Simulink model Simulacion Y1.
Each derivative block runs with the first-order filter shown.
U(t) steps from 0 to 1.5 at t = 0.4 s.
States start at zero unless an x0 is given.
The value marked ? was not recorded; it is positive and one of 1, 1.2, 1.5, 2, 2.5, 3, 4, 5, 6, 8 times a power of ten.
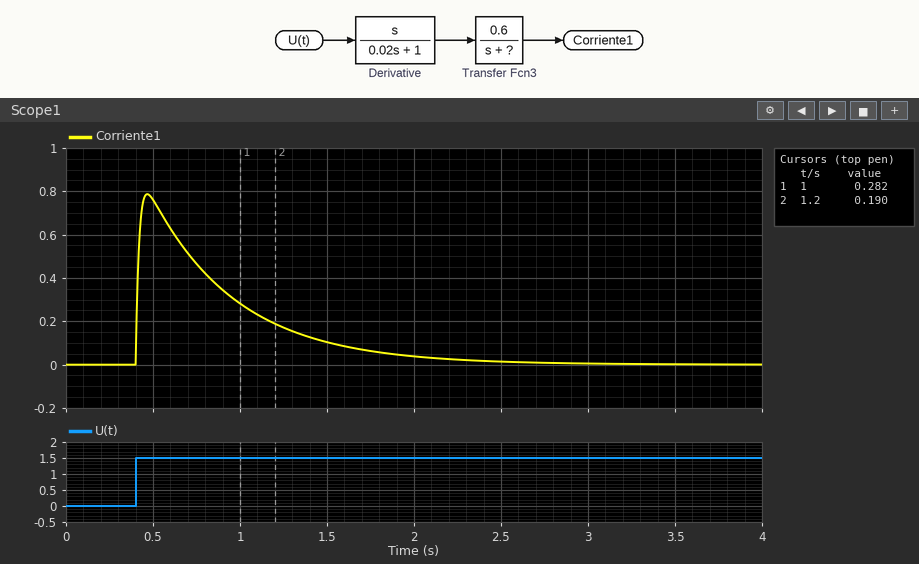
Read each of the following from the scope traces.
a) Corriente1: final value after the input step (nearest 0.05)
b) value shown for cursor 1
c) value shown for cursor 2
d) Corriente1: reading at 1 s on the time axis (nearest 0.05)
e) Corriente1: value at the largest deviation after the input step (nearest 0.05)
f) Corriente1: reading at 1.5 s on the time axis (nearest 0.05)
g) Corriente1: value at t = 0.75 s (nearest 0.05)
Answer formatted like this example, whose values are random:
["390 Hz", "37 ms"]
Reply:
["0.00", "0.282", "0.190", "0.30", "0.80", "0.10", "0.45"]
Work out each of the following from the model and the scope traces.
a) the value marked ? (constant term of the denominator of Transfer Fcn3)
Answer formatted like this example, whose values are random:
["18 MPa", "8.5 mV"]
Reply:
["2"]
